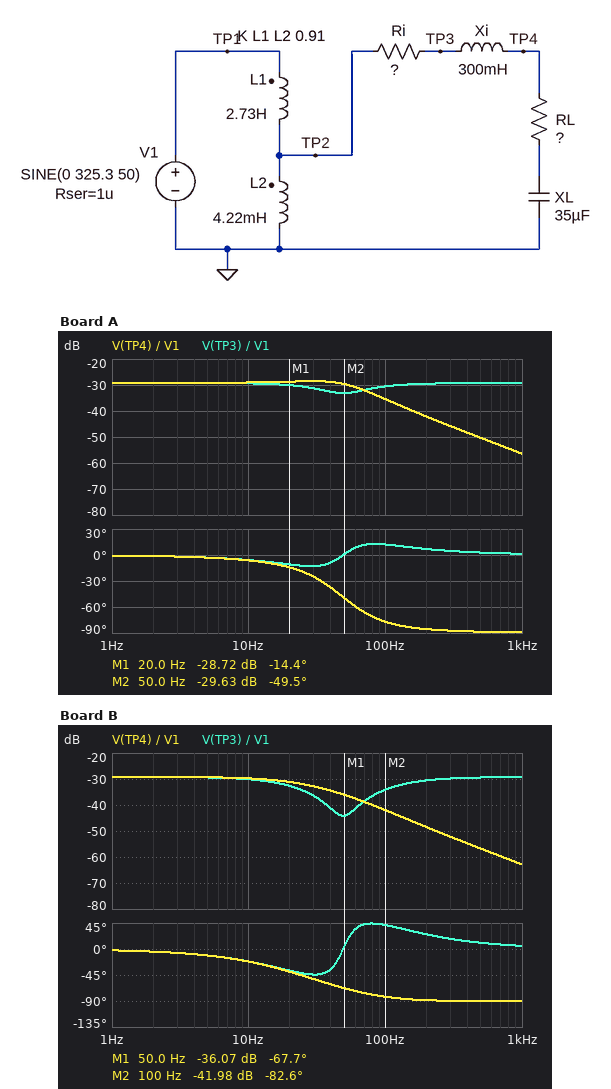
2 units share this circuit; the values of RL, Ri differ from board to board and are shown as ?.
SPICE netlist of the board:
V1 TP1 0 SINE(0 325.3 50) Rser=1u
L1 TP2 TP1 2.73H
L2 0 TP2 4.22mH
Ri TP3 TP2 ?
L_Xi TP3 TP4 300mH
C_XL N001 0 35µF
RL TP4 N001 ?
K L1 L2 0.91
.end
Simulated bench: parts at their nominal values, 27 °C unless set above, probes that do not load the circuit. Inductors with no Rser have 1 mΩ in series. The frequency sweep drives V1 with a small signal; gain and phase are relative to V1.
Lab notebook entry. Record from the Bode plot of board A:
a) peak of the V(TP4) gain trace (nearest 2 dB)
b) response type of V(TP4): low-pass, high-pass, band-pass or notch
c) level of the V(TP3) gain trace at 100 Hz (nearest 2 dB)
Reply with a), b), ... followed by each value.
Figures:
a) -28 dB
b) low-pass
c) -30 dB
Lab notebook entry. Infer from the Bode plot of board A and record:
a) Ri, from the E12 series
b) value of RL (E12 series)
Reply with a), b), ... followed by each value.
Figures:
a) 47 Ω
b) 82 Ω
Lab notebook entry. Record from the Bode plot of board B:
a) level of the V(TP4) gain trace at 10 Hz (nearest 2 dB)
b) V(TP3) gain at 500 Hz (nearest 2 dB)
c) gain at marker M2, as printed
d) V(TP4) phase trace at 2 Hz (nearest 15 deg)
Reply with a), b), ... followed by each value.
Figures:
a) -30 dB
b) -30 dB
c) -41.98 dB
d) 0 deg
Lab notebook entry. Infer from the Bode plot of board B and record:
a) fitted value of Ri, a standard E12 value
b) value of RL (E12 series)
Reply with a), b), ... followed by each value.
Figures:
a) 180 Ω
b) 39 Ω
